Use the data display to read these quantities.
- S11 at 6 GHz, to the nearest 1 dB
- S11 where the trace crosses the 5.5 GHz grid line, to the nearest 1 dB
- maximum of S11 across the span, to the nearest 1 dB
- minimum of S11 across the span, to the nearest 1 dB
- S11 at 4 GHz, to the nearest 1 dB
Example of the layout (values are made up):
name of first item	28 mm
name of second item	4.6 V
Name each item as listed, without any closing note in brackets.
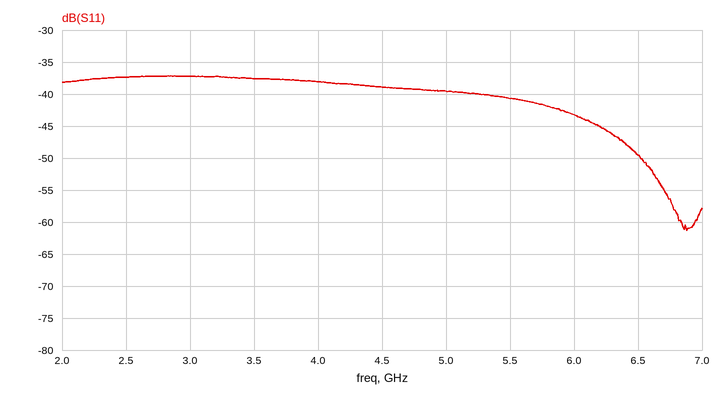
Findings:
S11 at 6 GHz, to the nearest 1 dB	-43 dB
S11 where the trace crosses the 5.5 GHz grid line, to the nearest 1 dB	-41 dB
maximum of S11 across the span, to the nearest 1 dB	-37 dB
minimum of S11 across the span, to the nearest 1 dB	-61 dB
S11 at 4 GHz, to the nearest 1 dB	-38 dB
